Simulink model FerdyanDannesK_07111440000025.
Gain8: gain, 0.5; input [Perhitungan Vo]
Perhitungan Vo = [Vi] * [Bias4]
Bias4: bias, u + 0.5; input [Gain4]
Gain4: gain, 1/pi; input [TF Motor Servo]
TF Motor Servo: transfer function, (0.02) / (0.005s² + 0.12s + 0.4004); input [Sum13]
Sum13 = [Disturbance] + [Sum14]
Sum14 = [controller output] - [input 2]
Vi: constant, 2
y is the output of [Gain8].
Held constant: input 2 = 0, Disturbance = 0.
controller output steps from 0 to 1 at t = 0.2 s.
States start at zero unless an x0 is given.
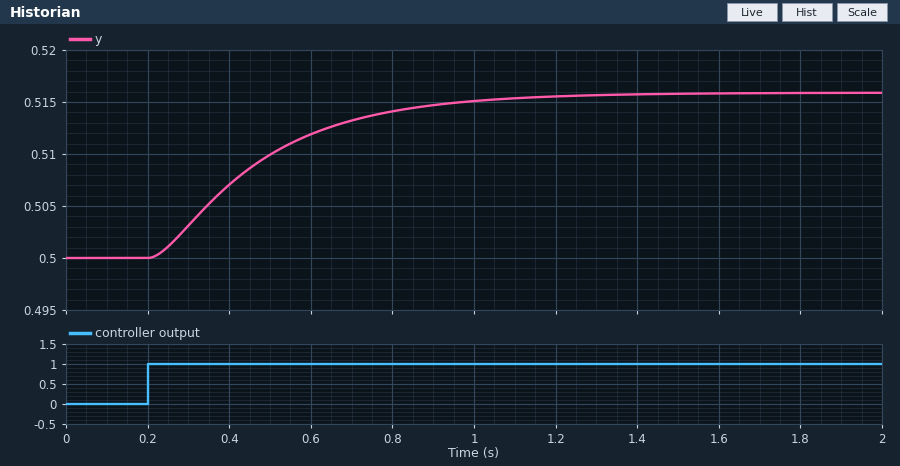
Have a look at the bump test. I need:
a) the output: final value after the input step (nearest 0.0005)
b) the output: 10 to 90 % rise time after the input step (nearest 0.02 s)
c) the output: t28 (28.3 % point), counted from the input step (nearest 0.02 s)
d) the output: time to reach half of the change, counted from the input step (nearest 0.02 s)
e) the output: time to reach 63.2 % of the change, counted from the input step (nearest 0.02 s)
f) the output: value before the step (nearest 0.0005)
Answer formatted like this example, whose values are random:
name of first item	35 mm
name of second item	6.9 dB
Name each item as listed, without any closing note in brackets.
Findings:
the output: final value after the input step	0.5160
the output: 10 to 90 % rise time after the input step	0.56 s
the output: t28 (28.3 % point), counted from the input step	0.14 s
the output: time to reach half of the change, counted from the input step	0.22 s
the output: time to reach 63.2 % of the change, counted from the input step	0.30 s
the output: value before the step	0.5000
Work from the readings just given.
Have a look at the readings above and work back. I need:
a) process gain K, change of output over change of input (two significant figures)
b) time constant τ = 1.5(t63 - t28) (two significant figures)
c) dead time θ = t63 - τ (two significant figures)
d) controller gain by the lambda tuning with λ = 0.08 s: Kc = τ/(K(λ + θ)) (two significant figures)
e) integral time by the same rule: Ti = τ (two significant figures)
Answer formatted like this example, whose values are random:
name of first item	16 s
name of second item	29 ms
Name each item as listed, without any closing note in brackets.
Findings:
process gain K, change of output over change of input	0.016
time constant τ = 1.5(t63 - t28)	0.24 s
dead time θ = t63 - τ	0.060 s
controller gain by the lambda tuning with λ = 0.08 s: Kc = τ/(K(λ + θ))	110
integral time by the same rule: Ti = τ	0.24 s
